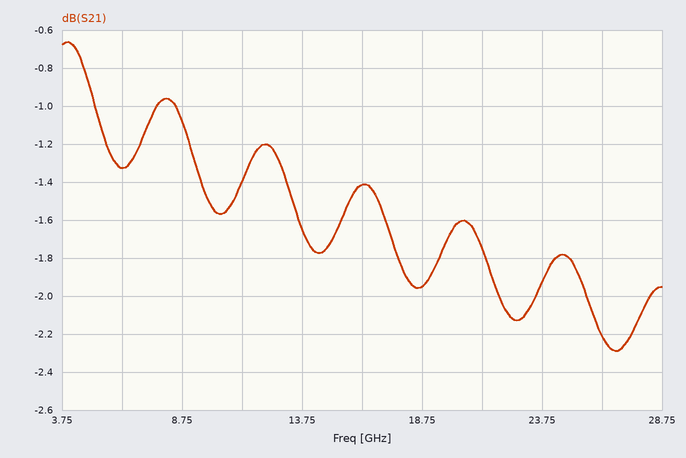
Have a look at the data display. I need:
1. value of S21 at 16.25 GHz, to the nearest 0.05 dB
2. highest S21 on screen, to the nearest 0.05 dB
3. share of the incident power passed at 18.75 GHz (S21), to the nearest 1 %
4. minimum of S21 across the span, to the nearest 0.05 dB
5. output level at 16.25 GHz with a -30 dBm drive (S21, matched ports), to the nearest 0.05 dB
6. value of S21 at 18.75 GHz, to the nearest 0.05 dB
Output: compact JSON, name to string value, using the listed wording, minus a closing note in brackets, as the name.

{"value of S21 at 16.25 GHz, to the nearest 0.05 dB": "-1.40 dB", "highest S21 on screen, to the nearest 0.05 dB": "-0.65 dB", "share of the incident power passed at 18.75 GHz (S21), to the nearest 1 %": "64 %", "minimum of S21 across the span, to the nearest 0.05 dB": "-2.30 dB", "output level at 16.25 GHz with a -30 dBm drive (S21, matched ports), to the nearest 0.05 dB": "-31.40 dBm", "value of S21 at 18.75 GHz, to the nearest 0.05 dB": "-1.95 dB"}
